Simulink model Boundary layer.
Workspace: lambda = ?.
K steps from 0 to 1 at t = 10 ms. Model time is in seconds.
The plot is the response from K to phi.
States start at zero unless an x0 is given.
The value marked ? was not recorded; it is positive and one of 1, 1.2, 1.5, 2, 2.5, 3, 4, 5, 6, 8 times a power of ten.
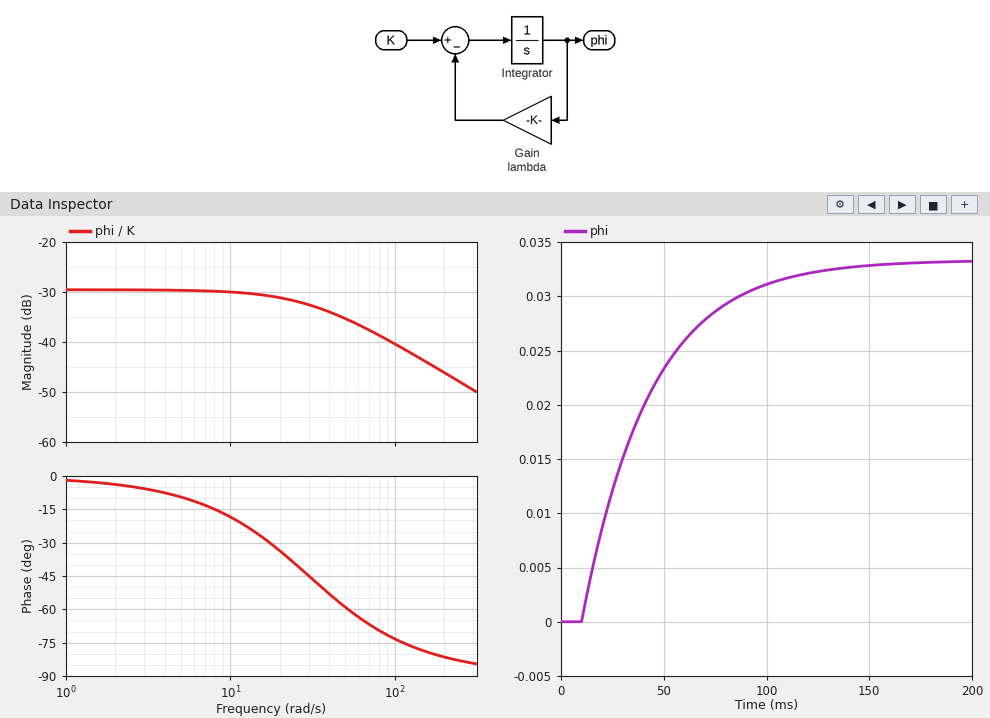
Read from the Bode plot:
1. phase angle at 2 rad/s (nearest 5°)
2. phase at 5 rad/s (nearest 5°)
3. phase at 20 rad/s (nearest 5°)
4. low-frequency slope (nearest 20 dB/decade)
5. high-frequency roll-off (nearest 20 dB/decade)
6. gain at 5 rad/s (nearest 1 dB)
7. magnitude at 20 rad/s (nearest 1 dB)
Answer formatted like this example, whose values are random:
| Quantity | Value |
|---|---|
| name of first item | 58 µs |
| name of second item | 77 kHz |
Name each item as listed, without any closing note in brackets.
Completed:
| Quantity | Value |
|---|---|
| phase angle at 2 rad/s | -5° |
| phase at 5 rad/s | -10° |
| phase at 20 rad/s | -35° |
| low-frequency slope | 0 dB/decade |
| high-frequency roll-off | -20 dB/decade |
| gain at 5 rad/s | -30 dB |
| magnitude at 20 rad/s | -31 dB |
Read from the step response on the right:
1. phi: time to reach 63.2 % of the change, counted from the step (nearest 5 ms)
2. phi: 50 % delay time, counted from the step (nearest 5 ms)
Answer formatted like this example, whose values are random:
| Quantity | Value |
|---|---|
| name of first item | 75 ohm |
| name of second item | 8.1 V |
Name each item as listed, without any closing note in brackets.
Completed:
| Quantity | Value |
|---|---|
| phi: time to reach 63.2 % of the change, counted from the step | 35 ms |
| phi: 50 % delay time, counted from the step | 25 ms |
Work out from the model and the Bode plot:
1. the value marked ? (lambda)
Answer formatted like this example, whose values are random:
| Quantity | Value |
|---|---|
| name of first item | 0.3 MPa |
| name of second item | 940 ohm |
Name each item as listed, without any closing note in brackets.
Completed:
| Quantity | Value |
|---|---|
| the value marked ? | 30 |
